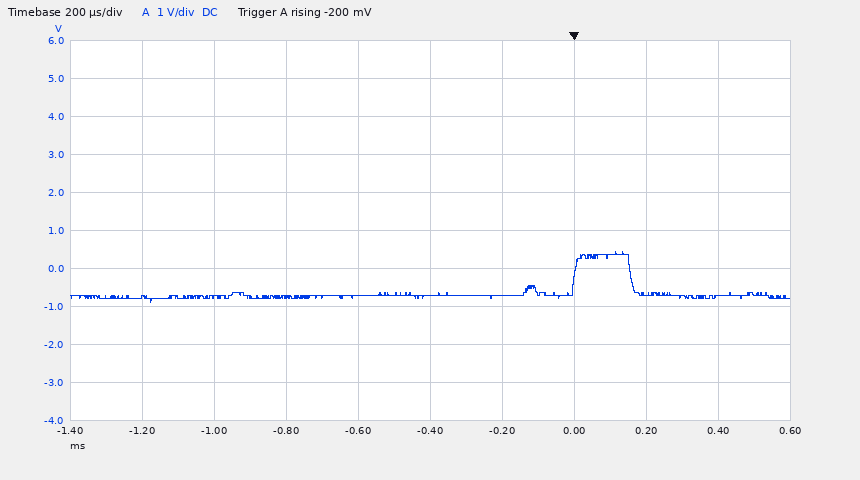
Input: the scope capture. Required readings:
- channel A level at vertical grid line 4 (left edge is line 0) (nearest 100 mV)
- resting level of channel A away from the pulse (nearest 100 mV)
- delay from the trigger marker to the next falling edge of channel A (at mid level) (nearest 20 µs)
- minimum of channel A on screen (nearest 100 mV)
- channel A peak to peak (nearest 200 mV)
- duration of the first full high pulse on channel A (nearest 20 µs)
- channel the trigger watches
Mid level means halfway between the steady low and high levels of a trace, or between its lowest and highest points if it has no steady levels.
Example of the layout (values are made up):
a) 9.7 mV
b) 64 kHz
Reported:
a) -700 mV
b) -700 mV
c) 160 µs
d) -900 mV
e) 1.4 V
f) 160 µs
g) channel A
